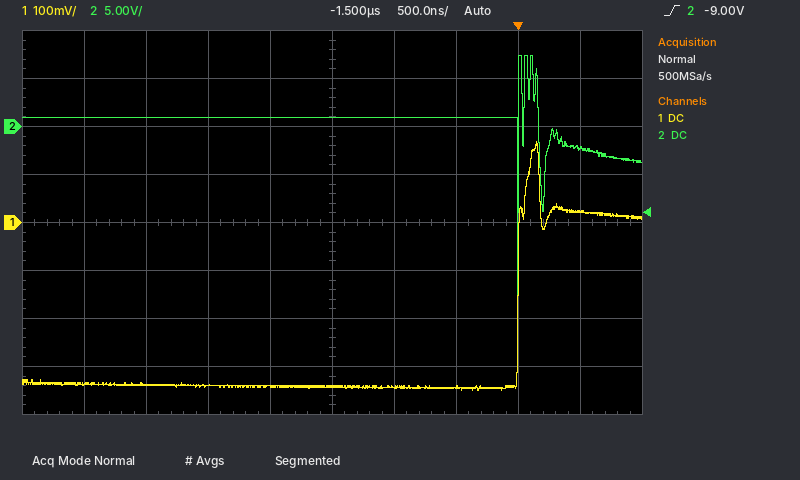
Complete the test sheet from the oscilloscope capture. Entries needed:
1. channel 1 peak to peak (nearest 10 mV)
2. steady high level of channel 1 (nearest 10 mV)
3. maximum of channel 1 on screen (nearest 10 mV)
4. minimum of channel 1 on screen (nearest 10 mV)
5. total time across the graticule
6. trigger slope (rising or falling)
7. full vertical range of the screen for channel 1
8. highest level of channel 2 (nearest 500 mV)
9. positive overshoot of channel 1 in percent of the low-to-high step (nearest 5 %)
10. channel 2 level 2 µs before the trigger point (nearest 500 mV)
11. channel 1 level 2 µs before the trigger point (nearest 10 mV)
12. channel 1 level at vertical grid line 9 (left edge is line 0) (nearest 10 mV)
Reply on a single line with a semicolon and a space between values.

520 mV; 20 mV; 170 mV; -350 mV; 5 µs; rising; 800 mV; 7.5 V; 40 %; 1.0 V; -340 mV; 20 mV
